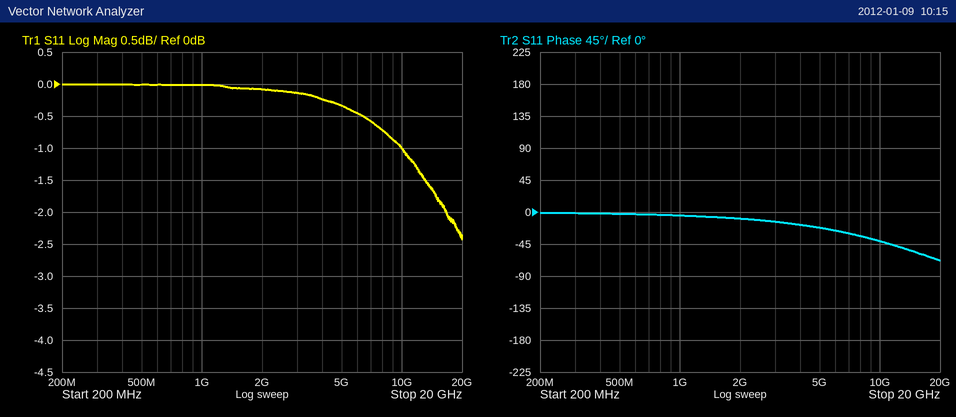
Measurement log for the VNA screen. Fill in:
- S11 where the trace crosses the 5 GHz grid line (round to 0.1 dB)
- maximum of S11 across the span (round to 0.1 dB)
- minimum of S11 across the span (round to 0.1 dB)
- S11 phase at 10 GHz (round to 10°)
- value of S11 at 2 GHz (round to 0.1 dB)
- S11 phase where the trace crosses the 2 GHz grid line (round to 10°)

-0.3 dB
0.0 dB
-2.4 dB
-40°
-0.1 dB
-10°
